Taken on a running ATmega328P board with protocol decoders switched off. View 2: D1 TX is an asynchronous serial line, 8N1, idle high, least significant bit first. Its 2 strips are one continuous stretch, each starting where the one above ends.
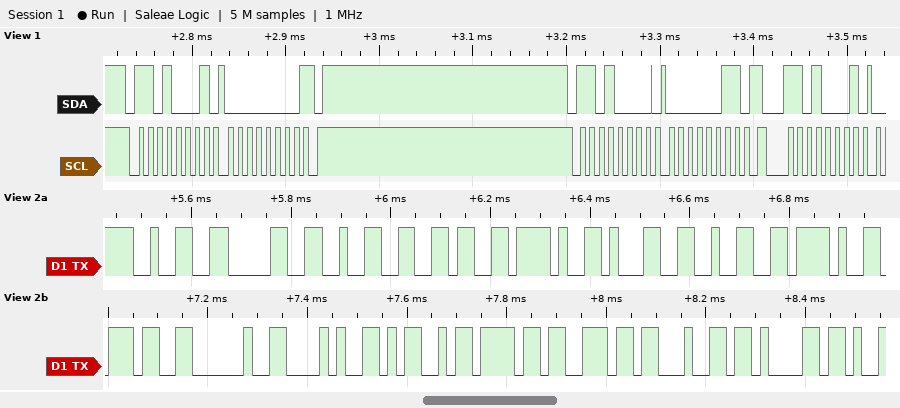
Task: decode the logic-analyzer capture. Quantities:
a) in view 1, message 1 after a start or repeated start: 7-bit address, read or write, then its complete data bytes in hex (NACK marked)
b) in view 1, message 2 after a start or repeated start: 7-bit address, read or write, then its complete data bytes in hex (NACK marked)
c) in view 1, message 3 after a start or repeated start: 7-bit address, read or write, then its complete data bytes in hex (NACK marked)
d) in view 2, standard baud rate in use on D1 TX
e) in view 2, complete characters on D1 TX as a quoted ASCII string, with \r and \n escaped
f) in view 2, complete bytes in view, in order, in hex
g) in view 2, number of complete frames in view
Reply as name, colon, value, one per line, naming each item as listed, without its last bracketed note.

in view 1, message 1 after a start or repeated start: 7-bit address, read or write, then its complete data bytes in hex: 0x68 read: 00 NACK
in view 1, message 2 after a start or repeated start: 7-bit address, read or write, then its complete data bytes in hex: 0x68 write: 03
in view 1, message 3 after a start or repeated start: 7-bit address, read or write, then its complete data bytes in hex: 0x68 read
in view 2, standard baud rate in use on D1 TX: 57600 baud
in view 2, complete characters on D1 TX as a quoted ASCII string, with \r and \n escaped: "2026/12/7 (Monda"
in view 2, complete bytes in view, in order, in hex: 0x32 0x30 0x32 0x36 0x2F 0x31 0x32 0x2F 0x37 0x20 0x28 0x4D 0x6F 0x6E 0x64 0x61
in view 2, number of complete frames in view: 16
